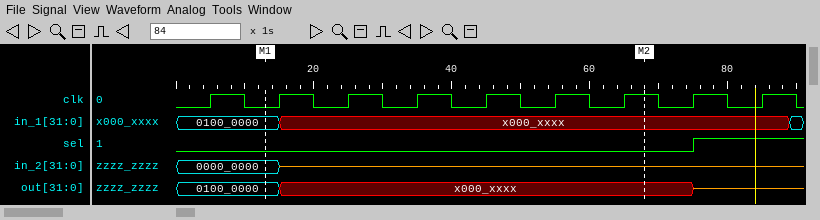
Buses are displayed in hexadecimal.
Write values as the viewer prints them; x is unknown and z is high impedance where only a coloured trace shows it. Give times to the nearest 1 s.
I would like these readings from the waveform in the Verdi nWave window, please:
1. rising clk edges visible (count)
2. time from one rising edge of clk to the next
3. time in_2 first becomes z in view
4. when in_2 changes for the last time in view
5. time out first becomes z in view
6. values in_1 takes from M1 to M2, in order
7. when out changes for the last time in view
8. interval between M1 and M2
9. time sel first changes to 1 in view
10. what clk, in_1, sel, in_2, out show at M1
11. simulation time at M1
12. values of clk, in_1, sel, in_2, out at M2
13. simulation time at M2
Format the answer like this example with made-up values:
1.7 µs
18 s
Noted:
9
10 s
15 s
15 s
75 s
0100_0000, x000_xxxx
75 s
55 s
75 s
clk=0, in_1=0100_0000, sel=0, in_2=0000_0000, out=0100_0000
13 s
clk=1, in_1=x000_xxxx, sel=0, in_2=z, out=x000_xxxx
68 s
